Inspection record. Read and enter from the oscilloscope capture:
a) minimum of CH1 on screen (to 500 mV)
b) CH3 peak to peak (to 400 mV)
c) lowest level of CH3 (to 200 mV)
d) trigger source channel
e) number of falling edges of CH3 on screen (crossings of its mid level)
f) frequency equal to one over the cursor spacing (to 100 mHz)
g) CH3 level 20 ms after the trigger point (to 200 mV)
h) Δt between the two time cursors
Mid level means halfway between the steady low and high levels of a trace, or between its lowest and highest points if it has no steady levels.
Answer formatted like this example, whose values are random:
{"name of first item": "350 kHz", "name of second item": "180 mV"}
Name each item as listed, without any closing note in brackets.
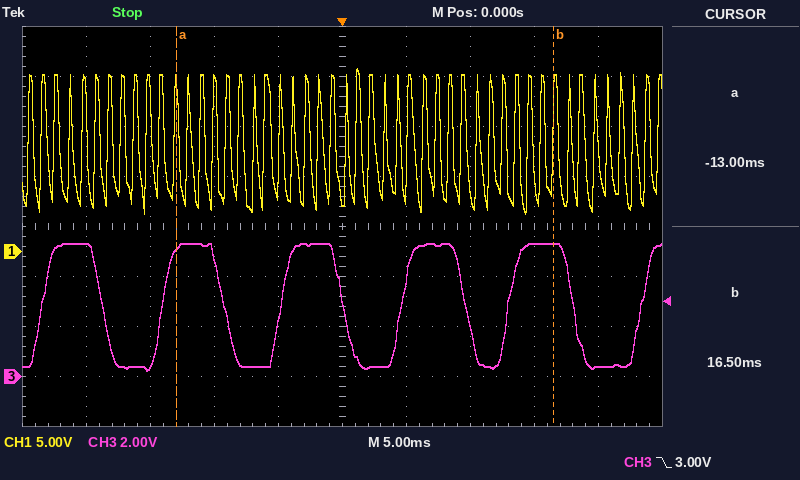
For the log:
{"minimum of CH1 on screen": "4.0 V", "CH3 peak to peak": "5.2 V", "lowest level of CH3": "200 mV", "trigger source channel": "CH3", "number of falling edges of CH3 on screen": "5", "frequency equal to one over the cursor spacing": "33.9 Hz", "CH3 level 20 ms after the trigger point": "400 mV", "Δt between the two time cursors": "29.5 ms"}
